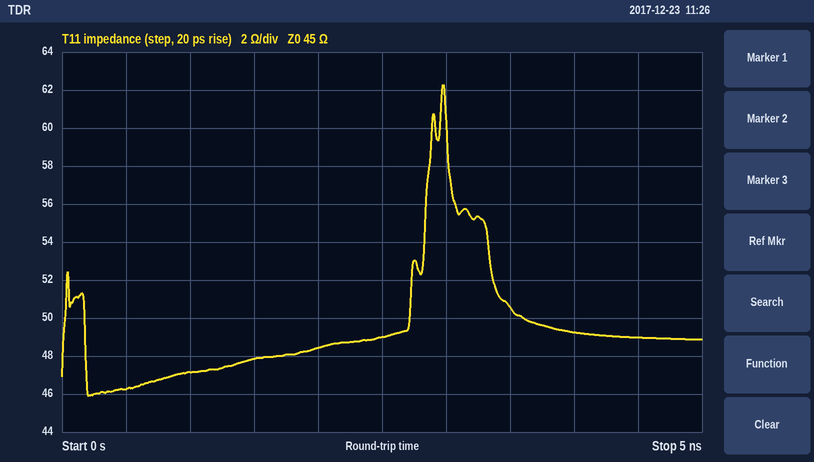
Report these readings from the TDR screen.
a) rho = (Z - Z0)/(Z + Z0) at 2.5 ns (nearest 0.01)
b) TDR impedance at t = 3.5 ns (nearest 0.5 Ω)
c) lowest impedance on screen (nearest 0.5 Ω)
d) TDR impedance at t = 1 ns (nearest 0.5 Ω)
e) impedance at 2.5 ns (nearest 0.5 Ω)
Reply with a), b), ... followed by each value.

a) +0.04
b) 50.5 Ω
c) 46.0 Ω
d) 47.0 Ω
e) 49.0 Ω
